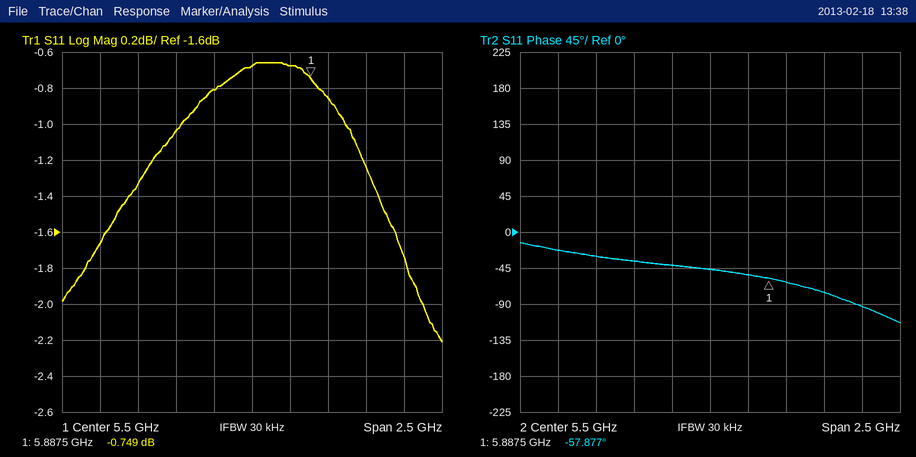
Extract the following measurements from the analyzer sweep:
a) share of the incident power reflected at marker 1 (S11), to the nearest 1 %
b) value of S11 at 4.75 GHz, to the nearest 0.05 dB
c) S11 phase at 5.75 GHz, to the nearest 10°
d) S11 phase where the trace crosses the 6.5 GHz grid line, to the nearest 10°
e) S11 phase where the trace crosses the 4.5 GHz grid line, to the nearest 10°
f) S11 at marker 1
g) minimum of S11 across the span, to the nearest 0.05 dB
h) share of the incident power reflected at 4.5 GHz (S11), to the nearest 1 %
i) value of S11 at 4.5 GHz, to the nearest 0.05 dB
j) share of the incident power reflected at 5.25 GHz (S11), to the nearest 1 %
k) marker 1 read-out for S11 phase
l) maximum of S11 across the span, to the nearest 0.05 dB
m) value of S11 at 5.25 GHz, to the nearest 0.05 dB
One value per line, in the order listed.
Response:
84 %
-1.35 dB
-50°
-90°
-20°
-0.749 dB
-2.20 dB
68 %
-1.65 dB
83 %
-57.877°
-0.65 dB
-0.80 dB
